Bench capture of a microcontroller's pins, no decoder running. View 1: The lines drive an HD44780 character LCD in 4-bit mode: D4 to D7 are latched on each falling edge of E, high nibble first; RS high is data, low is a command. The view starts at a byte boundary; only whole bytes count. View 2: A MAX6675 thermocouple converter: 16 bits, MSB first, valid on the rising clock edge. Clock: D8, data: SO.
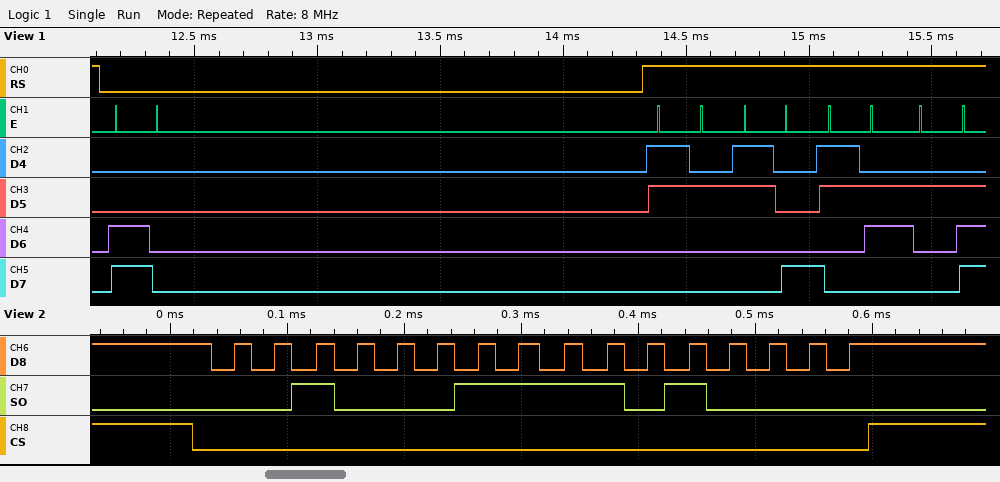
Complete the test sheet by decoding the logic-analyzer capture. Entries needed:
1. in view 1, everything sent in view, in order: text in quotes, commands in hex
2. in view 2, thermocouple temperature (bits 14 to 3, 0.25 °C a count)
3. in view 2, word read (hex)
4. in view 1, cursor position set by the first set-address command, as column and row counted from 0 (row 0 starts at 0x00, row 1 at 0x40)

0xC0 "286."
286.50 °C
0x23D0
column 0, row 1
